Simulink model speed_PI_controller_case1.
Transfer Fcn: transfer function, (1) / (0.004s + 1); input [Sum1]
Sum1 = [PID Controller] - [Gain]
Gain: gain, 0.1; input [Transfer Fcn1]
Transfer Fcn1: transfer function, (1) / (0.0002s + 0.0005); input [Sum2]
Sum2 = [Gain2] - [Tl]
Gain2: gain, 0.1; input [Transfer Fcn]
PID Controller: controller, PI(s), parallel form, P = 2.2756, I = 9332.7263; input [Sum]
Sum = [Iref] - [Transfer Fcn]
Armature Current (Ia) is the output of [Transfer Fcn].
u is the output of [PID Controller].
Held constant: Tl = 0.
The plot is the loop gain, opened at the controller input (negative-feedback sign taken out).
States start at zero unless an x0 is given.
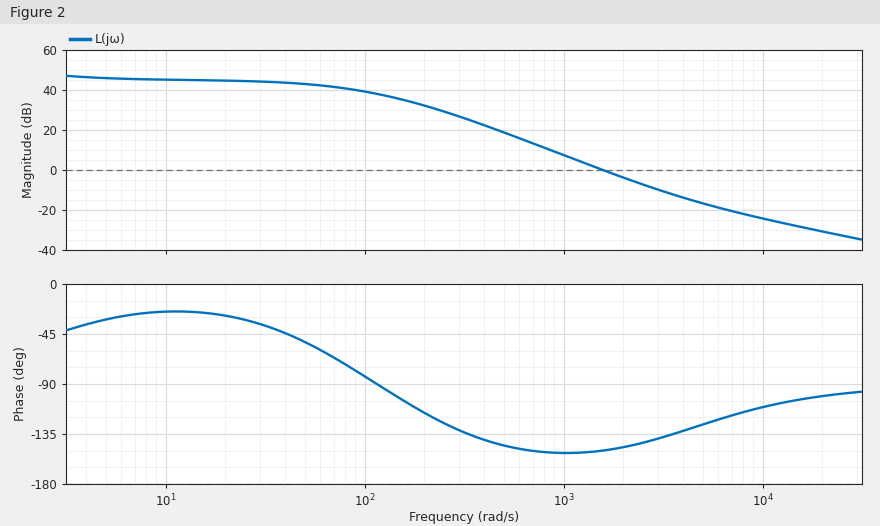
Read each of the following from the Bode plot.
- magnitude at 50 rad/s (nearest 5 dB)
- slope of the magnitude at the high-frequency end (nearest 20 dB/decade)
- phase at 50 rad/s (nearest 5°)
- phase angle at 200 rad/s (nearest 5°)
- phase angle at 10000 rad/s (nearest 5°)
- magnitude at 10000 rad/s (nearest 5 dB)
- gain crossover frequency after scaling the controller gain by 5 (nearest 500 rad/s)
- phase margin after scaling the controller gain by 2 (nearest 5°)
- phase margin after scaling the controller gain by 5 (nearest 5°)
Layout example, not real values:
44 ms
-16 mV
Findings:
45 dB
-20 dB/decade
-50°
-115°
-110°
-25 dB
4000 rad/s
35°
50°
